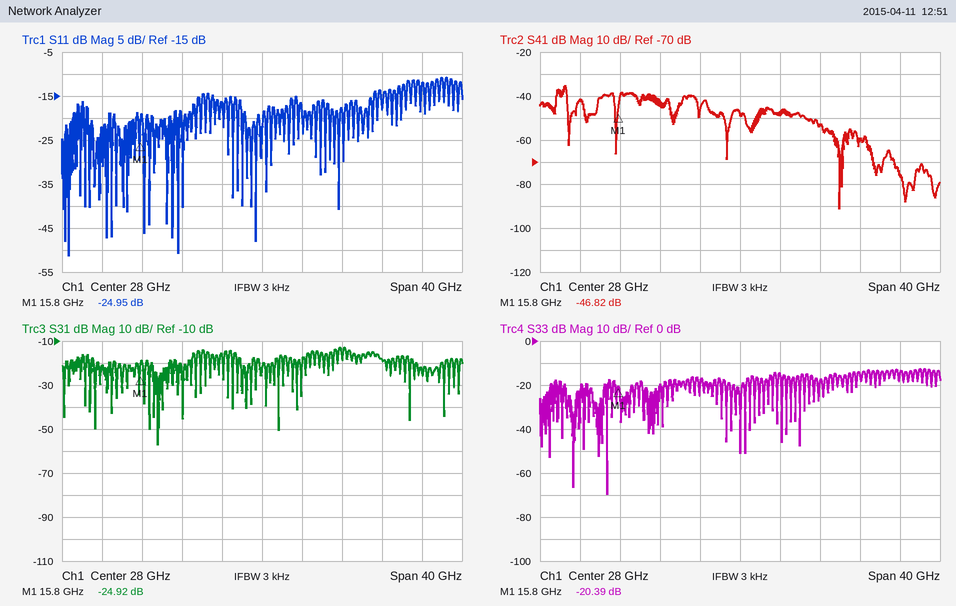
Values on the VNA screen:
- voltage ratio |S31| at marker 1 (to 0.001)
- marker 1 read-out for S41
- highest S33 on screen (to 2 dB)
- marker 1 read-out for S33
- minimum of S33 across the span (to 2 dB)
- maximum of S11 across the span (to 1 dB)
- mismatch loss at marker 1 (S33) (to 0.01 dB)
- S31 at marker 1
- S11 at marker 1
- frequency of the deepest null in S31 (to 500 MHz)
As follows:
0.057
-46.82 dB
-12 dB
-20.39 dB
-70 dB
-11 dB
0.04 dB
-24.92 dB
-24.95 dB
17.5 GHz
